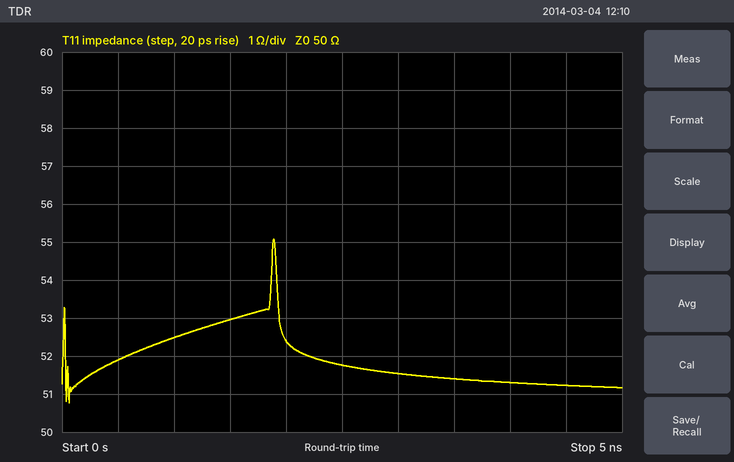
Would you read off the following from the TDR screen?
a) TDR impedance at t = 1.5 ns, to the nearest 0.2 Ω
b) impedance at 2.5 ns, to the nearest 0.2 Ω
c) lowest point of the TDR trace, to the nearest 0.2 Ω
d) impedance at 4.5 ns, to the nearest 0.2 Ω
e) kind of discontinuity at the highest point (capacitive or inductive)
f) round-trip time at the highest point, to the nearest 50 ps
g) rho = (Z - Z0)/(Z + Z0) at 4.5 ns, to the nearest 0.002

53.0 Ω
51.8 Ω
50.8 Ω
51.2 Ω
inductive
1.90 ns
+0.012
